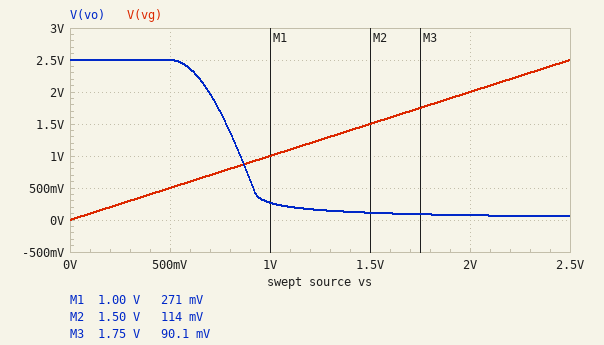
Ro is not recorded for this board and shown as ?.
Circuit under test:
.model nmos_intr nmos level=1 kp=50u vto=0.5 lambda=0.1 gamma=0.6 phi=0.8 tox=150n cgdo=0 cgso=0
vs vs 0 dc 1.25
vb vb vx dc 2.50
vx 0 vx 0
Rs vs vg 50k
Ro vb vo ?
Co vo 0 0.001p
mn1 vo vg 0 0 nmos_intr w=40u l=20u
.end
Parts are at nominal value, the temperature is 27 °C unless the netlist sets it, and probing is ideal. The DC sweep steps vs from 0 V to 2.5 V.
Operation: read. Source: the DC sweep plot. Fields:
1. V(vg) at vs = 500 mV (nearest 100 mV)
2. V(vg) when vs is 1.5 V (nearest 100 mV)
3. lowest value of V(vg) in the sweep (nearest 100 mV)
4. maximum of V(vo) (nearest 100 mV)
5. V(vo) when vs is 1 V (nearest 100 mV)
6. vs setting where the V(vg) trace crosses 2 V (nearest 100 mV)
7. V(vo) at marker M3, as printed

500 mV
1.5 V
0 V
2.5 V
300 mV
2.0 V
90.1 mV
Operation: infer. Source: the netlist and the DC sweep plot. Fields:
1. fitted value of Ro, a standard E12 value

220 kΩ
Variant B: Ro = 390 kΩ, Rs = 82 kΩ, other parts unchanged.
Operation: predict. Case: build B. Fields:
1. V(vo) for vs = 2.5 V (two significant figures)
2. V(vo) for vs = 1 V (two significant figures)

32 mV
140 mV
